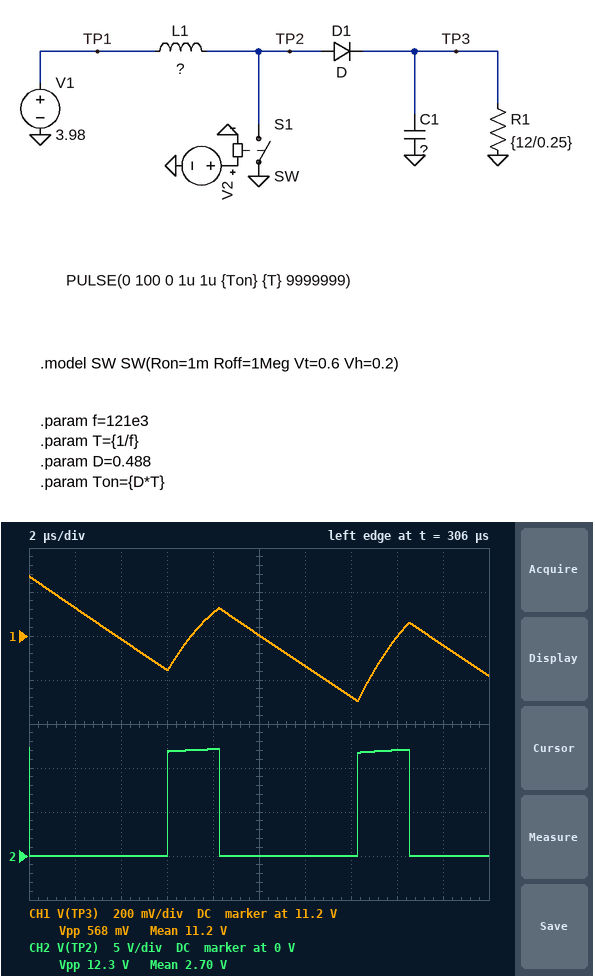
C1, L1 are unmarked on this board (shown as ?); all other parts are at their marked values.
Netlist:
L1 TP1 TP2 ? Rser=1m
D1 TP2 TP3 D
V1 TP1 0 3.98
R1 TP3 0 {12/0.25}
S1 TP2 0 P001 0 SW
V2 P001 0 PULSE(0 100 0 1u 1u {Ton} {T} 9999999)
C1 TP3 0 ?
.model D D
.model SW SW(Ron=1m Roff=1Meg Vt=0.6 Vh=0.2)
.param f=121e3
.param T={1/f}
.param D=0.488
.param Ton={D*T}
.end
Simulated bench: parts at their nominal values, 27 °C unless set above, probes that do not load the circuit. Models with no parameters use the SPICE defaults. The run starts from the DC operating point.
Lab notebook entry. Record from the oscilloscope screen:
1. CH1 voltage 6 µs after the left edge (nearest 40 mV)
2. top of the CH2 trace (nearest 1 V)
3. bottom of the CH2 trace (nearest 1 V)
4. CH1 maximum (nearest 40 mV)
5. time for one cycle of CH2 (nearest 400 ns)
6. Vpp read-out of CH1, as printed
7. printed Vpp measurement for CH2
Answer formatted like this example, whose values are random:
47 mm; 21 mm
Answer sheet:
11.04 V; 12 V; 0 V; 11.48 V; 8.4 µs; 568 mV; 12.3 V
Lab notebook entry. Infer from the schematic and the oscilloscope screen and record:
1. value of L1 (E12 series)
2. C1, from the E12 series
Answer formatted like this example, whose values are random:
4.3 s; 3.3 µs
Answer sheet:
56 µH; 3.3 µF
